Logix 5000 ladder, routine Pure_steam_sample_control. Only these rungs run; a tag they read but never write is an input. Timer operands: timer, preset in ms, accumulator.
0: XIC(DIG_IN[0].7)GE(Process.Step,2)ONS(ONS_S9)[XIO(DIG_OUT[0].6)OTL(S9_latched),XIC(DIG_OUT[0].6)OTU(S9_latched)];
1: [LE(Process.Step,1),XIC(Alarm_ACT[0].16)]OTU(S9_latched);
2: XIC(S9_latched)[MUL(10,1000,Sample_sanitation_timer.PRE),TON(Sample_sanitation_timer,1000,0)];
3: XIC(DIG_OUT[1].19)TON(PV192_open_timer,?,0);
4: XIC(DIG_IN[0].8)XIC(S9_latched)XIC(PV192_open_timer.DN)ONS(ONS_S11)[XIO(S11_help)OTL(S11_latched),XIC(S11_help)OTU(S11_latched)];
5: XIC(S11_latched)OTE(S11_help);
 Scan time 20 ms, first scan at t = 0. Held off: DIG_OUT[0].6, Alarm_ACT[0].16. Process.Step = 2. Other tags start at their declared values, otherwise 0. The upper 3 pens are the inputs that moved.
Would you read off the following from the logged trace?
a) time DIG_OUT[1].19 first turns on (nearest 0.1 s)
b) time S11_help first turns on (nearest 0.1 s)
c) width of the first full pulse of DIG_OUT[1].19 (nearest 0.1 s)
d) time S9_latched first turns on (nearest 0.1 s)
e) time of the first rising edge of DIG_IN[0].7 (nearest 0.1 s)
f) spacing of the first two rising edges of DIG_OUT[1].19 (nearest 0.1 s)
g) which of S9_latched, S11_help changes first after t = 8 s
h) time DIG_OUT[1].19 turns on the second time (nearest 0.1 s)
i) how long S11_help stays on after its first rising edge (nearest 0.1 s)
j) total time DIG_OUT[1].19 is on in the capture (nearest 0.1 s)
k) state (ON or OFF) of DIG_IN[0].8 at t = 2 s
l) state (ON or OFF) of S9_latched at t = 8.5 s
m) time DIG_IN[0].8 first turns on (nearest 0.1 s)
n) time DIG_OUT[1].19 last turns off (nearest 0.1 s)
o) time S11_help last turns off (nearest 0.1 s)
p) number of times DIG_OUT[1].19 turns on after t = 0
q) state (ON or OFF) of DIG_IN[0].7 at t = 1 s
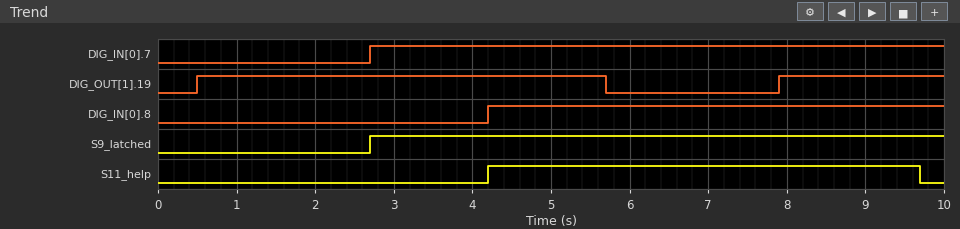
0.5 s
4.2 s
5.2 s
2.7 s
2.7 s
7.4 s
S11_help
7.9 s
5.5 s
7.3 s
OFF
ON
4.2 s
5.7 s
9.7 s
2
OFF
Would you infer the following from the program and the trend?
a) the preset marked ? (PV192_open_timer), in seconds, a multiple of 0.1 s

1.8 s
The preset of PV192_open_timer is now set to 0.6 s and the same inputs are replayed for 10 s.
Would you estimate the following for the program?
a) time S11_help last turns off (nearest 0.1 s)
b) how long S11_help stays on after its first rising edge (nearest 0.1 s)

8.5 s
4.3 s
